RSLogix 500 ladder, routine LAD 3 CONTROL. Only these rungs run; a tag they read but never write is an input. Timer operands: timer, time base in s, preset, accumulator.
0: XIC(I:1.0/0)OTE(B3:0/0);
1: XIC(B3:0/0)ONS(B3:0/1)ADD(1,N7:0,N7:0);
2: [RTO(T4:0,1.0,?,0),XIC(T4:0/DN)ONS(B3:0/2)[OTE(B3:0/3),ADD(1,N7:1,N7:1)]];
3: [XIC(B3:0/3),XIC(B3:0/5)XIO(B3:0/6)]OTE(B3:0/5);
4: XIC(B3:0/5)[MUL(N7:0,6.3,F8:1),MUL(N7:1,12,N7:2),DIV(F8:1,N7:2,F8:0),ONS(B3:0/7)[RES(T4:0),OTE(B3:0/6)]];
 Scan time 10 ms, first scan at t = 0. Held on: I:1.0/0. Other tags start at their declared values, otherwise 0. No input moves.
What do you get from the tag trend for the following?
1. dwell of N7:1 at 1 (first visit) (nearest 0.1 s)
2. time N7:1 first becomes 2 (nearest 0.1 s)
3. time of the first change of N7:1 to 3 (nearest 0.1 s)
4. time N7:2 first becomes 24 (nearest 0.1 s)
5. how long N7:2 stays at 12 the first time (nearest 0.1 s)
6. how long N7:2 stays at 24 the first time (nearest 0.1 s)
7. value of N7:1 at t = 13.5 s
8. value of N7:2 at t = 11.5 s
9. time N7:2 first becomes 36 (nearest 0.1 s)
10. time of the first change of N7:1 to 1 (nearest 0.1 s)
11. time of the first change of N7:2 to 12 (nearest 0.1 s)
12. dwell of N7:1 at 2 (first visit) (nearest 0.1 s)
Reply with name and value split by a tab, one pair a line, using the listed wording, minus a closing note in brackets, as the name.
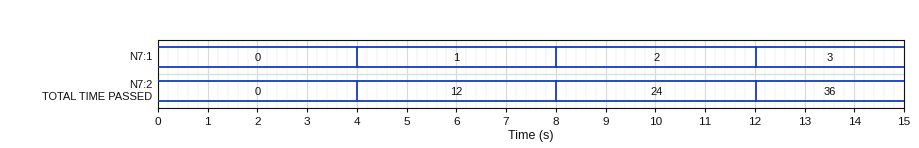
dwell of N7:1 at 1 (first visit)	4.0 s
time N7:1 first becomes 2	8.0 s
time of the first change of N7:1 to 3	12.0 s
time N7:2 first becomes 24	8.0 s
how long N7:2 stays at 12 the first time	4.0 s
how long N7:2 stays at 24 the first time	4.0 s
value of N7:1 at t = 13.5 s	3
value of N7:2 at t = 11.5 s	24
time N7:2 first becomes 36	12.0 s
time of the first change of N7:1 to 1	4.0 s
time of the first change of N7:2 to 12	4.0 s
dwell of N7:1 at 2 (first visit)	4.0 s
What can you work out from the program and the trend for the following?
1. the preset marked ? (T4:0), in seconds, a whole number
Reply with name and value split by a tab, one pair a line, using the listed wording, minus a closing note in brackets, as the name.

the preset marked ? (T4:0), in seconds, a whole number	4 s
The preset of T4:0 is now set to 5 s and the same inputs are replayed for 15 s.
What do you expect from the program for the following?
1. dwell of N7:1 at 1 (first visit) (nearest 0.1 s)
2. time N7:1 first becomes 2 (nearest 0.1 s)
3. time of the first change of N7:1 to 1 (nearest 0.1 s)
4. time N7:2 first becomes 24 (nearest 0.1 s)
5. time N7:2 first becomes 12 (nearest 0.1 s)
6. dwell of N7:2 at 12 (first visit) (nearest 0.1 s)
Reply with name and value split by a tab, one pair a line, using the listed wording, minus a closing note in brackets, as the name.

dwell of N7:1 at 1 (first visit)	5.0 s
time N7:1 first becomes 2	10.0 s
time of the first change of N7:1 to 1	5.0 s
time N7:2 first becomes 24	10.0 s
time N7:2 first becomes 12	5.0 s
dwell of N7:2 at 12 (first visit)	5.0 s
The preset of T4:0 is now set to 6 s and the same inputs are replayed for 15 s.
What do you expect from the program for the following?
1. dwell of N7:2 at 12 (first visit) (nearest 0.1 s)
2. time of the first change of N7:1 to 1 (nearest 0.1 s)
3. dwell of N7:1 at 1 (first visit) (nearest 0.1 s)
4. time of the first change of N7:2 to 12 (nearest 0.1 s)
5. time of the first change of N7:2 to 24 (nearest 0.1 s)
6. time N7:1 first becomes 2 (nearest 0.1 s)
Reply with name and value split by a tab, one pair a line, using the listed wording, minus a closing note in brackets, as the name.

dwell of N7:2 at 12 (first visit)	6.0 s
time of the first change of N7:1 to 1	6.0 s
dwell of N7:1 at 1 (first visit)	6.0 s
time of the first change of N7:2 to 12	6.0 s
time of the first change of N7:2 to 24	12.0 s
time N7:1 first becomes 2	12.0 s
